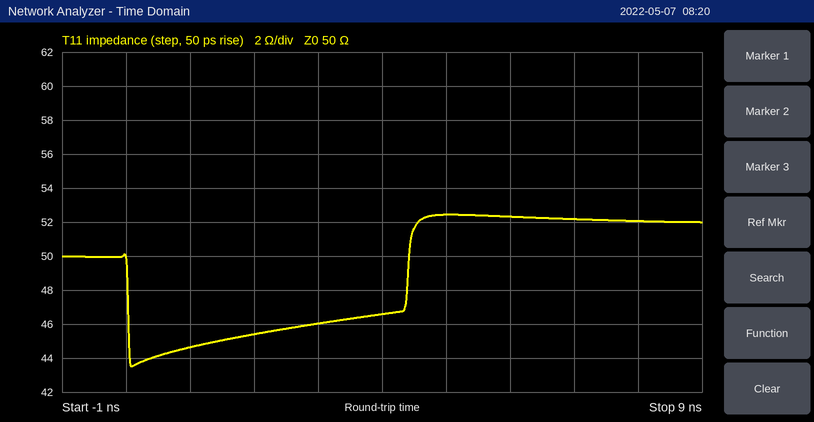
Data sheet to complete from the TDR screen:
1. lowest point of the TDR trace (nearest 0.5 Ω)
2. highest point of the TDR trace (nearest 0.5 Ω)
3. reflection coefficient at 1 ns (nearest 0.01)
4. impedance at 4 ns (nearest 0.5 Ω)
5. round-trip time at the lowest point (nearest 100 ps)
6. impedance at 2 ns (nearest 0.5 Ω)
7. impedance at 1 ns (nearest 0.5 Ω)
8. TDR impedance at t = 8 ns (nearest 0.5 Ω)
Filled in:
43.5 Ω
52.5 Ω
-0.06
46.5 Ω
100 ps
45.5 Ω
44.5 Ω
52.0 Ω
